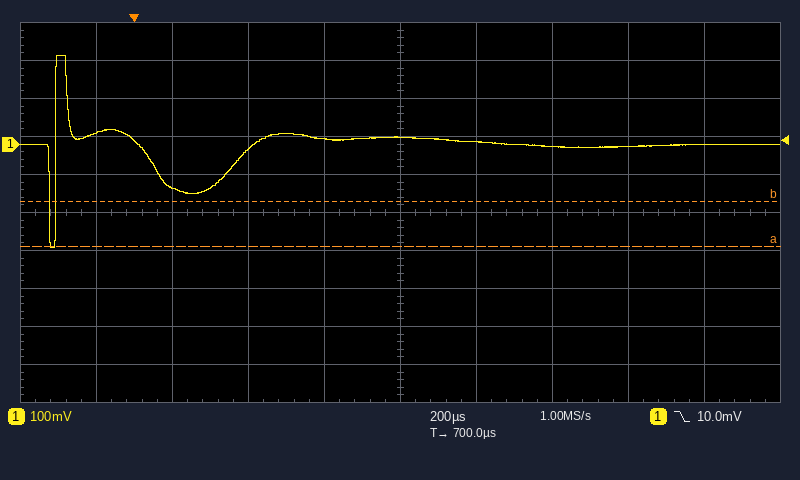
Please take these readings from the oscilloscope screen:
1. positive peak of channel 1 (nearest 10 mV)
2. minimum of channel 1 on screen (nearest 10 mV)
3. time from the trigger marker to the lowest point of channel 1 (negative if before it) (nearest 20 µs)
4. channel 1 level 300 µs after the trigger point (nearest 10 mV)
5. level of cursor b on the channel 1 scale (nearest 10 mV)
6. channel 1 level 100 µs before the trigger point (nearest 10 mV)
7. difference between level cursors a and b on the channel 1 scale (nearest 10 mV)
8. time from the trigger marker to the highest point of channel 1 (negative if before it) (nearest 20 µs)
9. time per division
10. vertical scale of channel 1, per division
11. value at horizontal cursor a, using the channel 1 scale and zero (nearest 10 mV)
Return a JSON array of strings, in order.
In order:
["230 mV", "-270 mV", "-220 µs", "-10 mV", "-150 mV", "30 mV", "120 mV", "-200 µs", "200 µs", "100 mV", "-270 mV"]
